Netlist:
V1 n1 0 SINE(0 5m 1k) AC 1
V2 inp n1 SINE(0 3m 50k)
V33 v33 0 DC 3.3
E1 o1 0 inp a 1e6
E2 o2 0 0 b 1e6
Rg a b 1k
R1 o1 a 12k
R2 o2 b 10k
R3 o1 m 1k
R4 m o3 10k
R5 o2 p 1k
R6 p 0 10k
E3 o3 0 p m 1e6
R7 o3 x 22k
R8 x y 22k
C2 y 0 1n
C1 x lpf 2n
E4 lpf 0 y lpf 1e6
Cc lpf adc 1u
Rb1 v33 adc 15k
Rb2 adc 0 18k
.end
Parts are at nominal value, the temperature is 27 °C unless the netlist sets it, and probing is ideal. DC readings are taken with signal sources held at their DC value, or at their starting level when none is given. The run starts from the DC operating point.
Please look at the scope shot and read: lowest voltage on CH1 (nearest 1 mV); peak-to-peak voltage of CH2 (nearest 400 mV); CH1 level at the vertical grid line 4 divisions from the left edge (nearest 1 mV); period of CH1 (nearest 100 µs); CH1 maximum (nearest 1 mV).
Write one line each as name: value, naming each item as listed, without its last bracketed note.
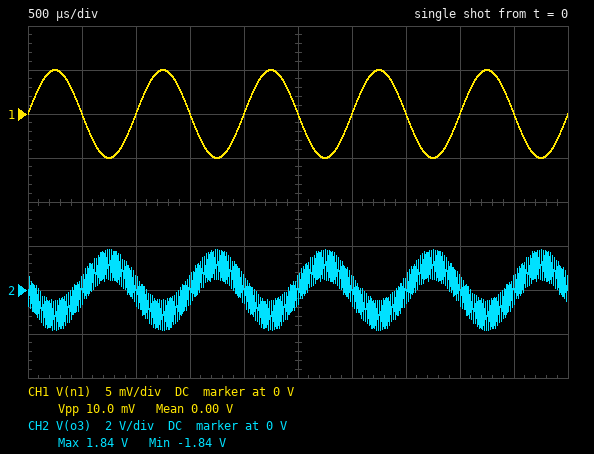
lowest voltage on CH1: -5 mV
peak-to-peak voltage of CH2: 3.6 V
CH1 level at the vertical grid line 4 divisions from the left edge: 0 V
period of CH1: 1.0 ms
CH1 maximum: 5 mV
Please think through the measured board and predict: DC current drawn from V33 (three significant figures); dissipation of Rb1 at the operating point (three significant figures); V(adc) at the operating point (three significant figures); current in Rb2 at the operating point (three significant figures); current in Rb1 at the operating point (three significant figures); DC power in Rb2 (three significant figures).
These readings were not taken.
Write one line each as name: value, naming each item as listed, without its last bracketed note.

DC current drawn from V33: 100 µA
dissipation of Rb1 at the operating point: 150 µW
V(adc) at the operating point: 1.80 V
current in Rb2 at the operating point: 100 µA
current in Rb1 at the operating point: 100 µA
DC power in Rb2: 180 µW
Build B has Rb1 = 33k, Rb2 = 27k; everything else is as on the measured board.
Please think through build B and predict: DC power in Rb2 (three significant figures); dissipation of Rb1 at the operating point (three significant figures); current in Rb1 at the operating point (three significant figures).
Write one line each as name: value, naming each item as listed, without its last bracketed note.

DC power in Rb2: 81.7 µW
dissipation of Rb1 at the operating point: 99.8 µW
current in Rb1 at the operating point: 55.0 µA
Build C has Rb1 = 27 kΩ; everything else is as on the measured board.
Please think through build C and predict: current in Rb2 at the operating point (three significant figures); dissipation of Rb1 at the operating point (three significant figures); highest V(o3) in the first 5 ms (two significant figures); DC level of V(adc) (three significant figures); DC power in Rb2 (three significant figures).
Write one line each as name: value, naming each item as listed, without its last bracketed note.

current in Rb2 at the operating point: 73.3 µA
dissipation of Rb1 at the operating point: 145 µW
highest V(o3) in the first 5 ms: 1.8 V
DC level of V(adc): 1.32 V
DC power in Rb2: 96.8 µW
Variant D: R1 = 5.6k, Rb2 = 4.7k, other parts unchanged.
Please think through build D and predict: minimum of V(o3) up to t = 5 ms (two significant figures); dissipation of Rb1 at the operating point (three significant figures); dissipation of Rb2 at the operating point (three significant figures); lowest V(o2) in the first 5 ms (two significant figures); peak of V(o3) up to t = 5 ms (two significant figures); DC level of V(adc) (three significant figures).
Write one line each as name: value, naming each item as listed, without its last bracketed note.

minimum of V(o3) up to t = 5 ms: -1.3 V
dissipation of Rb1 at the operating point: 421 µW
dissipation of Rb2 at the operating point: 132 µW
lowest V(o2) in the first 5 ms: -80 mV
peak of V(o3) up to t = 5 ms: 1.3 V
DC level of V(adc): 787 mV
